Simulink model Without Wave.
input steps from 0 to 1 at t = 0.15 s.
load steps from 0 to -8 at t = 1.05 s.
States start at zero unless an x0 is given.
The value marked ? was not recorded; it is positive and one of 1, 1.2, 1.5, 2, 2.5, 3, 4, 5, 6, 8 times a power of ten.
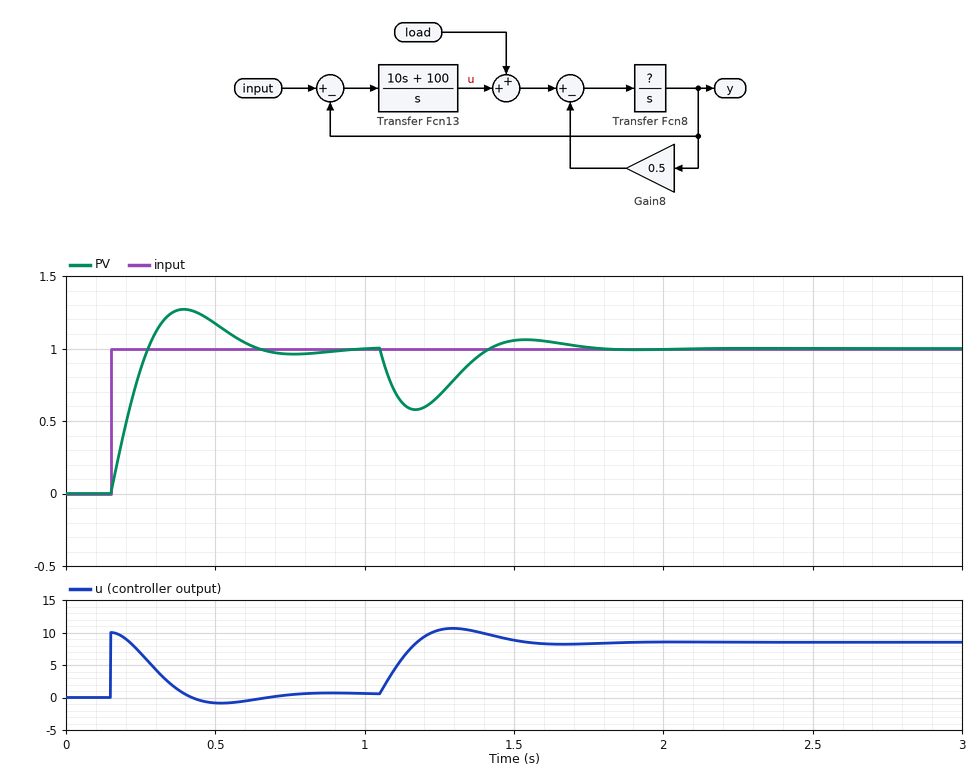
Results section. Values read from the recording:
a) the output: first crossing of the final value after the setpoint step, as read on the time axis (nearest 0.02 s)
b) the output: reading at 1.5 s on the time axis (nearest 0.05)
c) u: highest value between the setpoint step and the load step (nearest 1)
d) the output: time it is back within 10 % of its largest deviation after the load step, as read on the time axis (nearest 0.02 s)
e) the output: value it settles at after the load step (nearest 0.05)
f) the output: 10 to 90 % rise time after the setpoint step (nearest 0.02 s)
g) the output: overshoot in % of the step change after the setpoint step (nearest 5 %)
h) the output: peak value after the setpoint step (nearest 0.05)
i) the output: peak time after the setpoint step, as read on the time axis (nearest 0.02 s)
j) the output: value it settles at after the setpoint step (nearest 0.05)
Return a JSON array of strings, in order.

["0.28 s", "1.05", "10", "1.64 s", "1.00", "0.10 s", "25 %", "1.25", "0.40 s", "1.00"]
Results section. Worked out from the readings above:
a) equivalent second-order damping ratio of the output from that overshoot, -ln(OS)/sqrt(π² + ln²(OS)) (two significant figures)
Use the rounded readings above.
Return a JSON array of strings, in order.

["0.40"]
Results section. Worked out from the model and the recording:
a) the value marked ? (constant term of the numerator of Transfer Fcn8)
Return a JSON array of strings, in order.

["1"]
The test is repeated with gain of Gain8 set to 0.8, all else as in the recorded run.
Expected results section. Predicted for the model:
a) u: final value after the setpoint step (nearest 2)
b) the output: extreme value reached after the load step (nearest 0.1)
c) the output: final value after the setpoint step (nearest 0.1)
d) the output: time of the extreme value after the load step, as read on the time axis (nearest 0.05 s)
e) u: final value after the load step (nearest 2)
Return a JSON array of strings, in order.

["0", "0.6", "1.0", "1.15 s", "8"]
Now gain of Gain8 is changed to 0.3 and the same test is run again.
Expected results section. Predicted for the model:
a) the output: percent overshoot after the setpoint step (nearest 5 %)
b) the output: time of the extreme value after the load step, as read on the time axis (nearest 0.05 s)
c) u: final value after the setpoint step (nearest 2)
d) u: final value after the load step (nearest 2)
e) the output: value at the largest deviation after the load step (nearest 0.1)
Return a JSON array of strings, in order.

["30 %", "1.15 s", "0", "8", "0.6"]
